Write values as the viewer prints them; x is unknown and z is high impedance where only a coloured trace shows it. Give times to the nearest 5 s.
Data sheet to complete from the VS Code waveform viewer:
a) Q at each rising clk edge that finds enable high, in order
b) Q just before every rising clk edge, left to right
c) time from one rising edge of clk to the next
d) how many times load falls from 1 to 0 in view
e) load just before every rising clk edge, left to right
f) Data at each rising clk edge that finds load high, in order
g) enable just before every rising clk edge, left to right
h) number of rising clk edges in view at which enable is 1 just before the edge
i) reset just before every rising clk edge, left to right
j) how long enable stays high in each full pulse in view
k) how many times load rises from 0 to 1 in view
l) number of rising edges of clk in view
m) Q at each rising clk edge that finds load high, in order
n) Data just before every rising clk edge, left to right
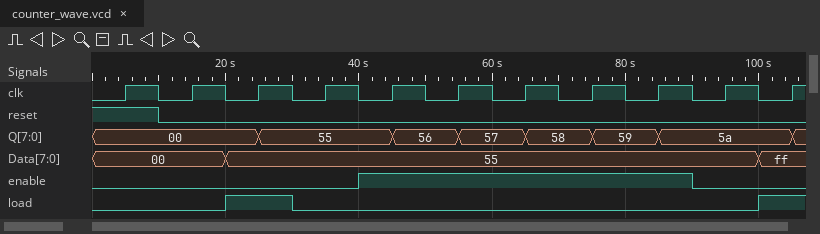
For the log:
55, 56, 57, 58, 59
00, 00, 00, 55, 55, 56, 57, 58, 59, 5a, 5a
10 s
1
0 0 1 0 0 0 0 0 0 0 1
55, ff
0 0 0 0 1 1 1 1 1 0 0
5
1 0 0 0 0 0 0 0 0 0 0
50 s
2
11
00, 5a
00, 00, 55, 55, 55, 55, 55, 55, 55, 55, ff
